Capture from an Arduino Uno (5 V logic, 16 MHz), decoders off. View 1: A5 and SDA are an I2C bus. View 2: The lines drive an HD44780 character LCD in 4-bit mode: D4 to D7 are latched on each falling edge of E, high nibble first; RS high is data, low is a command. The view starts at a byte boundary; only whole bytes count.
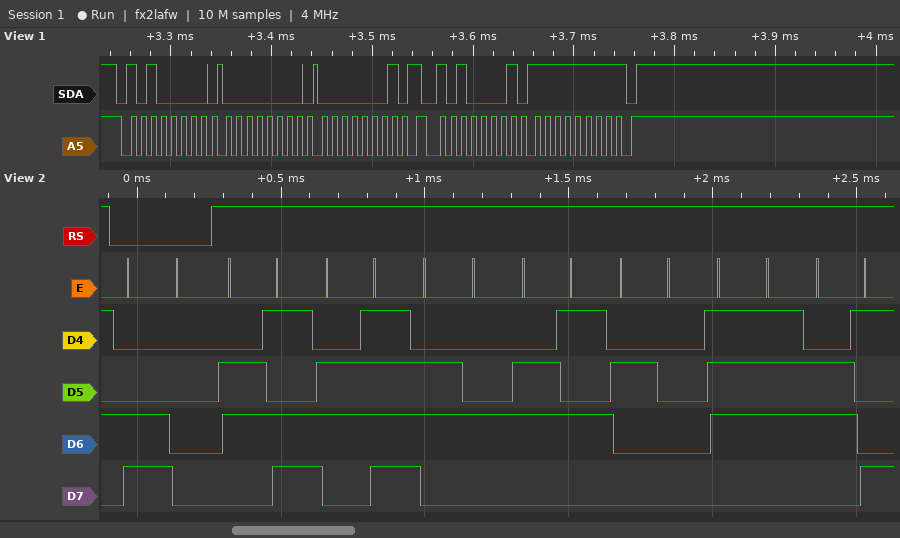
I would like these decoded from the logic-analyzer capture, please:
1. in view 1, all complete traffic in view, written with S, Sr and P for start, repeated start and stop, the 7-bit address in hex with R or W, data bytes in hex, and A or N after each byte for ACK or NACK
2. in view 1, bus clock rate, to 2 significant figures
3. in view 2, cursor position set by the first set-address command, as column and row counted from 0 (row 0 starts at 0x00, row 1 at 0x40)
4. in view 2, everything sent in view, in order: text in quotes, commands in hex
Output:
S 50W A 00 A 01 A Sr 50R A FF N P
100 kHz
column 0, row 1
0xC0 "mode wi"
